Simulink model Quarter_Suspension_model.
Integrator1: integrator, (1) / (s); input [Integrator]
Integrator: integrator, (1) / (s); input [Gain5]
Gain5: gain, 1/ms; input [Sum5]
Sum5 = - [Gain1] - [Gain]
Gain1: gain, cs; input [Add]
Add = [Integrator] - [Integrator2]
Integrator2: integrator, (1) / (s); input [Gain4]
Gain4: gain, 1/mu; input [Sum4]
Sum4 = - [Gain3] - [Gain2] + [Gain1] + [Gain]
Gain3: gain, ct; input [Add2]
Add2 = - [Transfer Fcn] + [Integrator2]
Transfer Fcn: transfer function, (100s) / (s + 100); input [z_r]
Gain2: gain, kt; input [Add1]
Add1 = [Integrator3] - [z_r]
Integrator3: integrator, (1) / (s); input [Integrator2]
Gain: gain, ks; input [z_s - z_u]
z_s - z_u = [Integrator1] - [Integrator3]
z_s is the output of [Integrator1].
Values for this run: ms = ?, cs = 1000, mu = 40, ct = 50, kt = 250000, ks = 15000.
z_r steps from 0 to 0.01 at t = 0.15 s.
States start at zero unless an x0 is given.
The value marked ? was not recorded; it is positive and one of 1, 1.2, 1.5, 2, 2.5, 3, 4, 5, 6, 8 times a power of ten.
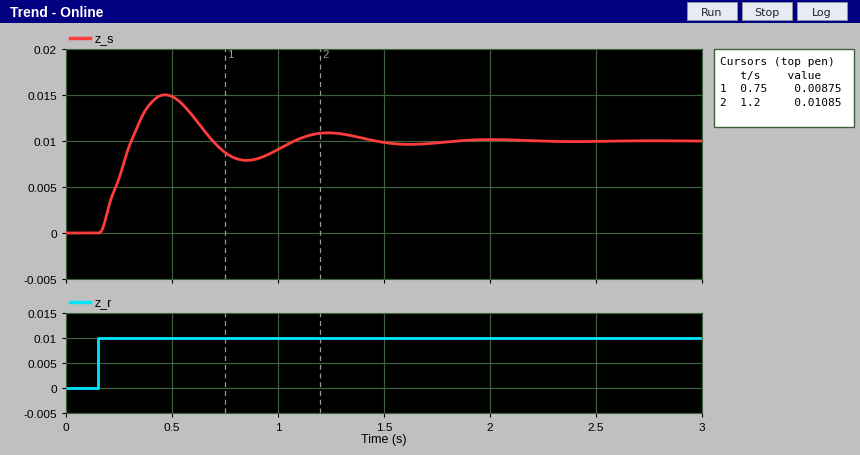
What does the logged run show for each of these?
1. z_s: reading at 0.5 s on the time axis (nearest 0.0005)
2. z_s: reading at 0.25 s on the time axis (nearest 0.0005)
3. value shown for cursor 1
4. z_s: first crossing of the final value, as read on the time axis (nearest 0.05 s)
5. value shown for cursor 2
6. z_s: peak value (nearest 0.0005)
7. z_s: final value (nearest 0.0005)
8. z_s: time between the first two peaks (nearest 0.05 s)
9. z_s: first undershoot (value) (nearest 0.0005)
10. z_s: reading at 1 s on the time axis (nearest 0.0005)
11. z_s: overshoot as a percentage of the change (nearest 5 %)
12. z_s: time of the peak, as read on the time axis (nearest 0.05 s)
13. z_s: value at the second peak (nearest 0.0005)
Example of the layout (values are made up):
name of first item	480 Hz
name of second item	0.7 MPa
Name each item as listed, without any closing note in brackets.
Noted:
z_s: reading at 0.5 s on the time axis	0.0150
z_s: reading at 0.25 s on the time axis	0.0060
value shown for cursor 1	0.00875
z_s: first crossing of the final value, as read on the time axis	0.30 s
value shown for cursor 2	0.01085
z_s: peak value	0.0150
z_s: final value	0.0100
z_s: time between the first two peaks	0.75 s
z_s: first undershoot (value)	0.0080
z_s: reading at 1 s on the time axis	0.0090
z_s: overshoot as a percentage of the change	50 %
z_s: time of the peak, as read on the time axis	0.45 s
z_s: value at the second peak	0.0110
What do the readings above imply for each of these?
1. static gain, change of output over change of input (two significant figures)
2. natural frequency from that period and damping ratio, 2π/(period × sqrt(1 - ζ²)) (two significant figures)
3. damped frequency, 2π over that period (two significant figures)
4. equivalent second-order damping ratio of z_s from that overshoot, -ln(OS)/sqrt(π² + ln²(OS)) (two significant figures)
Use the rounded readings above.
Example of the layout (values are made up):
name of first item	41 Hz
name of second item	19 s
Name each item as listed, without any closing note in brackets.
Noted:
static gain, change of output over change of input	1.0
natural frequency from that period and damping ratio, 2π/(period × sqrt(1 - ζ²))	8.6 rad/s
damped frequency, 2π over that period	8.4 rad/s
equivalent second-order damping ratio of z_s from that overshoot, -ln(OS)/sqrt(π² + ln²(OS))	0.22
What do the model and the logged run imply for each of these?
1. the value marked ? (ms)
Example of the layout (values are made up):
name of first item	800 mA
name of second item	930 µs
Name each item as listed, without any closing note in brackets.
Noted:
the value marked ?	200
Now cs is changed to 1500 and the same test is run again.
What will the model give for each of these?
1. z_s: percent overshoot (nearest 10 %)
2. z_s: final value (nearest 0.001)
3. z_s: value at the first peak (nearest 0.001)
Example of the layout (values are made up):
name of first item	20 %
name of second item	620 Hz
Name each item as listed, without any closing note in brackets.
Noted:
z_s: percent overshoot	40 %
z_s: final value	0.010
z_s: value at the first peak	0.014
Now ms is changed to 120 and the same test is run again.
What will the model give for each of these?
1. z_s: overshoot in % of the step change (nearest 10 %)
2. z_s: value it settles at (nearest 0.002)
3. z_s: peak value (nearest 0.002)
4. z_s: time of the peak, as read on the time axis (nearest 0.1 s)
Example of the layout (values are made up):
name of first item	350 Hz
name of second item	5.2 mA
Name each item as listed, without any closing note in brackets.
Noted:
z_s: overshoot in % of the step change	40 %
z_s: value it settles at	0.010
z_s: peak value	0.014
z_s: time of the peak, as read on the time axis	0.4 s
